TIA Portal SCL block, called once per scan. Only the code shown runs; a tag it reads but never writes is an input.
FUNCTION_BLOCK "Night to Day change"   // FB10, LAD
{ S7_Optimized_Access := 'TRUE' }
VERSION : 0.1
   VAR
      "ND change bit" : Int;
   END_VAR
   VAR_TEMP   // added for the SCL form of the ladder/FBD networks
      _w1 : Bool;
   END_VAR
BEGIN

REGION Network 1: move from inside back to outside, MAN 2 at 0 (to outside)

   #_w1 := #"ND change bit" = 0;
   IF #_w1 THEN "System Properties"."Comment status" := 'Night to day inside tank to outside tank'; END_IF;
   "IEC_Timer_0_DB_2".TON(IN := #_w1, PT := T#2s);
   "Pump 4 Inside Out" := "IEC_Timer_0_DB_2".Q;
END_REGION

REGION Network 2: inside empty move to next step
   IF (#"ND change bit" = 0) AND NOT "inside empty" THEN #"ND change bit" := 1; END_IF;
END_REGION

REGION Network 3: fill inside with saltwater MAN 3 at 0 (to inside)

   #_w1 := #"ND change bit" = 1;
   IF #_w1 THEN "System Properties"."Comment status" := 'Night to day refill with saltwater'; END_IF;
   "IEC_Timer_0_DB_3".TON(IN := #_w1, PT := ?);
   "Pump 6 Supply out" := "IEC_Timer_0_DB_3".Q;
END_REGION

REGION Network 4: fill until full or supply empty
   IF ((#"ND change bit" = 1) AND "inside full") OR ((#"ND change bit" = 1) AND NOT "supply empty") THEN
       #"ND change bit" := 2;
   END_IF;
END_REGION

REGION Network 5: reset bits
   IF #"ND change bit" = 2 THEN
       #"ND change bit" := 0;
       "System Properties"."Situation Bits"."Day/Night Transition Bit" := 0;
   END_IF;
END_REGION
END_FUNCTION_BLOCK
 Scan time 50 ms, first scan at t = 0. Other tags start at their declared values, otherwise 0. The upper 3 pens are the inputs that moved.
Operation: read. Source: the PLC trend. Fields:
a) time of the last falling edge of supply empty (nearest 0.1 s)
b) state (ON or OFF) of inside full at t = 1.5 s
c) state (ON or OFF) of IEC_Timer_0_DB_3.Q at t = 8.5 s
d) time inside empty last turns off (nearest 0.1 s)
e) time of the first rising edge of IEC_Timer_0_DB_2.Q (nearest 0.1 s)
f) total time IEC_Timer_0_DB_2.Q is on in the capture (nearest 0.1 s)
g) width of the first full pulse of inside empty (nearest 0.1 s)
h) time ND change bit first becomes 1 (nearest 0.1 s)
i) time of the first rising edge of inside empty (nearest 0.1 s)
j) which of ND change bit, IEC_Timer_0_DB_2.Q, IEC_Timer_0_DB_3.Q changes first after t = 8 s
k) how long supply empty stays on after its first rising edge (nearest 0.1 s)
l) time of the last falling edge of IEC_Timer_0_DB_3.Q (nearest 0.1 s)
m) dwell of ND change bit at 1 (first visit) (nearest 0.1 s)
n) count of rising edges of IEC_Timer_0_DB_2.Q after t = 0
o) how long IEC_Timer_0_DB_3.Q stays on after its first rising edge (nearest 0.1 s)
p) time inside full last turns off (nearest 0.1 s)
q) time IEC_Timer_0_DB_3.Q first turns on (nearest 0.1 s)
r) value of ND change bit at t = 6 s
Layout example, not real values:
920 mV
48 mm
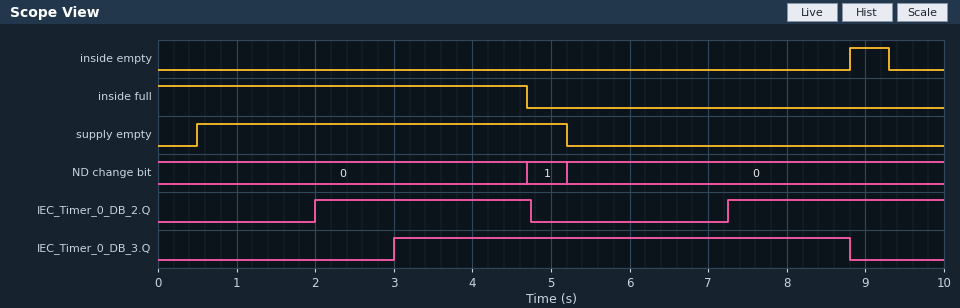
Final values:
5.2 s
ON
ON
9.3 s
2.0 s
5.5 s
0.5 s
4.7 s
8.8 s
IEC_Timer_0_DB_3.Q
4.7 s
8.8 s
0.5 s
2
5.8 s
4.7 s
3.0 s
0
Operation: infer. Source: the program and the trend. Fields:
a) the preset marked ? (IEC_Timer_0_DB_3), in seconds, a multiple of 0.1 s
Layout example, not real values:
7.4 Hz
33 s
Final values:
3.0 s
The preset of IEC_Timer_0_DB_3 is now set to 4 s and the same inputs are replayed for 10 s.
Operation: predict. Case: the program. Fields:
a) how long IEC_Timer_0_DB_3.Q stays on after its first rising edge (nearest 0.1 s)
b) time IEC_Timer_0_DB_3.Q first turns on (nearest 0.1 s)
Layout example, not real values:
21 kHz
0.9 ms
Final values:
4.8 s
4.0 s
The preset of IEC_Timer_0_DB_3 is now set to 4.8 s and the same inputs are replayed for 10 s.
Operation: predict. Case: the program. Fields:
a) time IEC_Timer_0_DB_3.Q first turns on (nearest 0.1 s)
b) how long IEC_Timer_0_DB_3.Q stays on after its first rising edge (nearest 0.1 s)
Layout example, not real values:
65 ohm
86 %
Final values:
4.8 s
4.0 s
